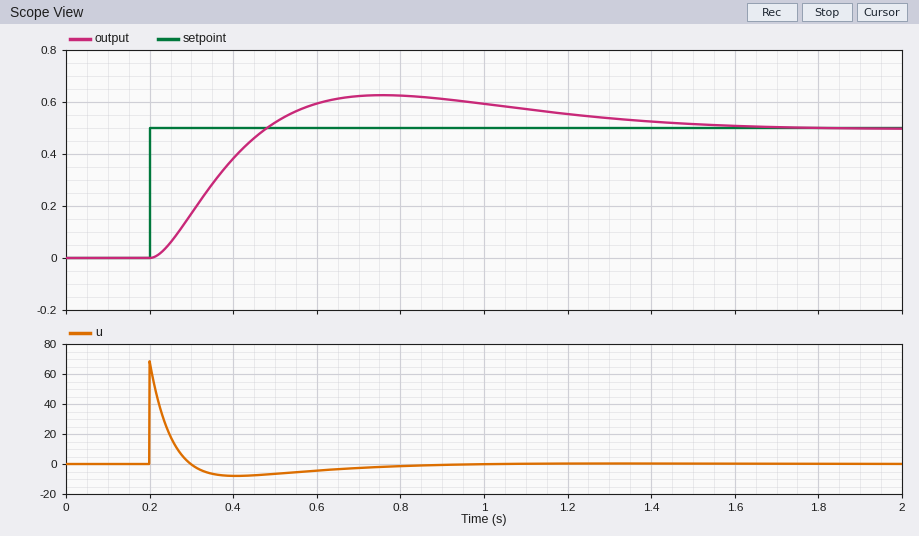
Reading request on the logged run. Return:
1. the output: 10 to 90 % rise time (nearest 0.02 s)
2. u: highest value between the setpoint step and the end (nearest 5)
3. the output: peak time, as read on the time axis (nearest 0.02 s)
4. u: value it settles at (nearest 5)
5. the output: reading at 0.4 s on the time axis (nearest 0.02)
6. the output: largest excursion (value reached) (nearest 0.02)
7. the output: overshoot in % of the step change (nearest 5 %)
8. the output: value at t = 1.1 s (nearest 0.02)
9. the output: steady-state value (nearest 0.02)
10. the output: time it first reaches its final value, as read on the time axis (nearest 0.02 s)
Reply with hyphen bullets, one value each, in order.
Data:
- 0.20 s
- 70
- 0.76 s
- 0
- 0.38
- 0.62
- 25 %
- 0.58
- 0.50
- 0.48 s
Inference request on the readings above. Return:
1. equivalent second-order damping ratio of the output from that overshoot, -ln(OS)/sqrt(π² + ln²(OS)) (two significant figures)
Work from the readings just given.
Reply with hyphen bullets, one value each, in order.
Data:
- 0.40
